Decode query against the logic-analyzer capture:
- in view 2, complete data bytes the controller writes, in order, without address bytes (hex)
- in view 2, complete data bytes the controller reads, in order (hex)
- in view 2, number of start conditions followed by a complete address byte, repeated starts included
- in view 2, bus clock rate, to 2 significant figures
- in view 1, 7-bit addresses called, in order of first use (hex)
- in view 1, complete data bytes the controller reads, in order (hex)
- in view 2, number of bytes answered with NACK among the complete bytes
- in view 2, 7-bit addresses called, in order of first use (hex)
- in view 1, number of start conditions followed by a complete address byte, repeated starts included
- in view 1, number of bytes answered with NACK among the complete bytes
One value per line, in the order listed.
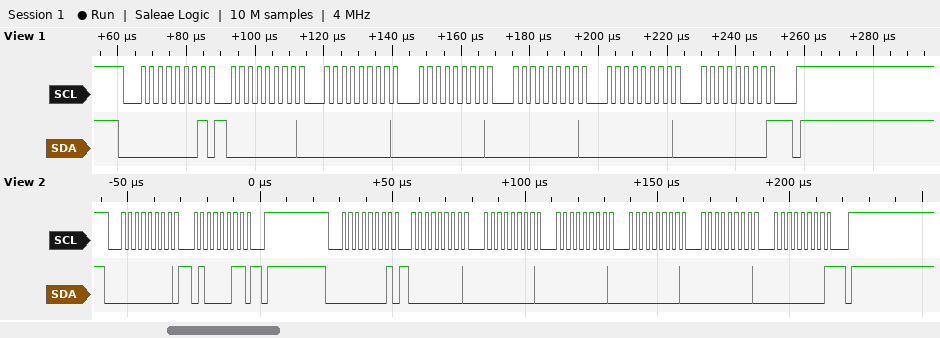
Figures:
43
00 00 00 00 00 00
2
400 kHz
0x00
00 00 00 00 00 00
1
0x00
1
1
